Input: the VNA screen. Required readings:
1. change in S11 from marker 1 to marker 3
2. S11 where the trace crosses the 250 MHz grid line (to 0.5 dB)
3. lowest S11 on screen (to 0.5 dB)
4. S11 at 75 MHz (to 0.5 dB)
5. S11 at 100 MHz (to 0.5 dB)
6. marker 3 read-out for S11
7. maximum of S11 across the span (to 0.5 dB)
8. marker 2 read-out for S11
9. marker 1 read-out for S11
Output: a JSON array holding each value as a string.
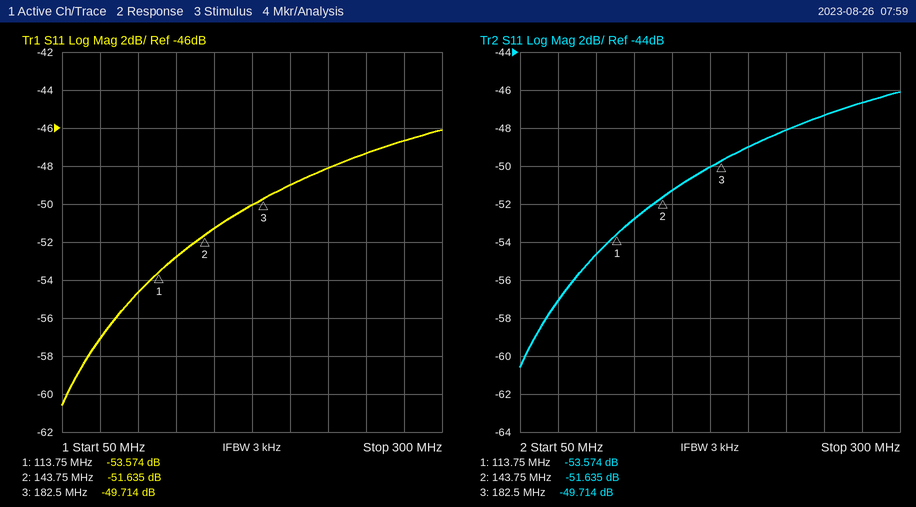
["3.860 dB", "-47.5 dB", "-60.5 dB", "-57.0 dB", "-54.5 dB", "-49.714 dB", "-46.0 dB", "-51.635 dB", "-53.574 dB"]
